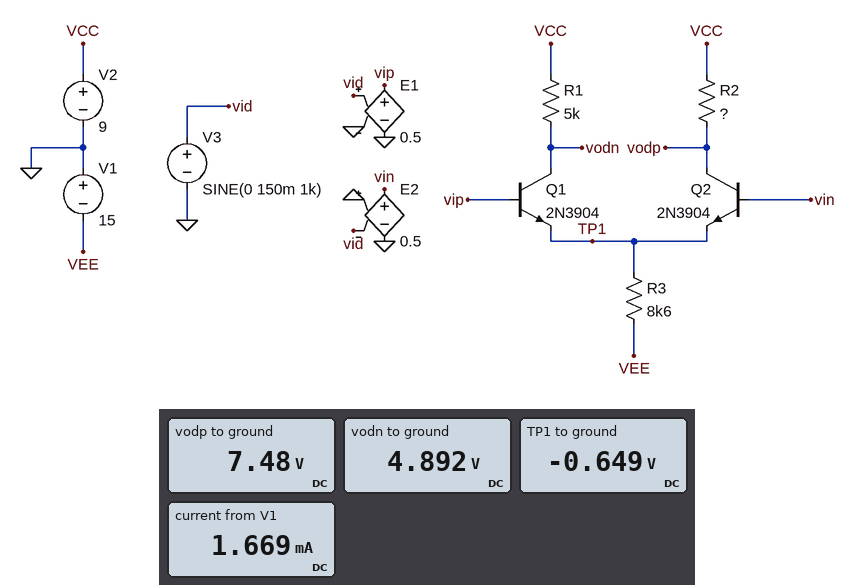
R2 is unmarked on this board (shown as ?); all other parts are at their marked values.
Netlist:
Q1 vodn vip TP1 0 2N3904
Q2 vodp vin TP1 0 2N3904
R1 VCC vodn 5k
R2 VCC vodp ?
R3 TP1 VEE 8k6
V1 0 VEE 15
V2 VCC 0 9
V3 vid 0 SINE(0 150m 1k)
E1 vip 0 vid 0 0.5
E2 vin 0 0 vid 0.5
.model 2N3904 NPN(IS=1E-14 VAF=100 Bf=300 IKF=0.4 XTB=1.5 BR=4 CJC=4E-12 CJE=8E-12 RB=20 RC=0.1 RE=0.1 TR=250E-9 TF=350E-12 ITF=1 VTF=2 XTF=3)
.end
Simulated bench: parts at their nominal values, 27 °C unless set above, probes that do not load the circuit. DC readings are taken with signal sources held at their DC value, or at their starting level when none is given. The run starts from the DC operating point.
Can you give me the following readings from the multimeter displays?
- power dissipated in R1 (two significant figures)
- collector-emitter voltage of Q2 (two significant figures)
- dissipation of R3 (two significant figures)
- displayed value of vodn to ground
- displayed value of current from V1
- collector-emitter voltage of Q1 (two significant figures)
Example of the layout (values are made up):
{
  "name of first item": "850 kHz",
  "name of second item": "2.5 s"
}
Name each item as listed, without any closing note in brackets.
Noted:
{
  "power dissipated in R1": "3.4 mW",
  "collector-emitter voltage of Q2": "8.1 V",
  "dissipation of R3": "24 mW",
  "displayed value of vodn to ground": "4.892 V",
  "displayed value of current from V1": "1.669 mA",
  "collector-emitter voltage of Q1": "5.5 V"
}
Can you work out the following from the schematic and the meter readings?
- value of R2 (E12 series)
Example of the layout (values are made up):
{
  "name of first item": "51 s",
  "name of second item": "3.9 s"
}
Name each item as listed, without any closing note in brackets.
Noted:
{
  "value of R2": "1.8 kΩ"
}
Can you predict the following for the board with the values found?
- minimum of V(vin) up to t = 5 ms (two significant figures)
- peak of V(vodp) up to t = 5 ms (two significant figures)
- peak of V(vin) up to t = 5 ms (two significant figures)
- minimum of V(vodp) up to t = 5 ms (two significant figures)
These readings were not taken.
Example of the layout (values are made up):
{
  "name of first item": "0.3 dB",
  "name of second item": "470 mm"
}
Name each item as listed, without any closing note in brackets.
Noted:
{
  "minimum of V(vin) up to t = 5 ms": "-75 mV",
  "peak of V(vodp) up to t = 5 ms": "9.0 V",
  "peak of V(vin) up to t = 5 ms": "75 mV",
  "minimum of V(vodp) up to t = 5 ms": "6.0 V"
}
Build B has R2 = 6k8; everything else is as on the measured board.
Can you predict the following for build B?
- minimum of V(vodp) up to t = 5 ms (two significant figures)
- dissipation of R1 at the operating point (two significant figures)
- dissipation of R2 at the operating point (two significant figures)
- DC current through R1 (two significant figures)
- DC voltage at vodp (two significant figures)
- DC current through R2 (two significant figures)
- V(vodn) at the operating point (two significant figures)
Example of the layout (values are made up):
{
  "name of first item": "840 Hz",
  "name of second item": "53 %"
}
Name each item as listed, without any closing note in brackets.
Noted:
{
  "minimum of V(vodp) up to t = 5 ms": "-600 mV",
  "dissipation of R1 at the operating point": "3.5 mW",
  "dissipation of R2 at the operating point": "4.6 mW",
  "DC current through R1": "840 µA",
  "DC voltage at vodp": "3.4 V",
  "DC current through R2": "830 µA",
  "V(vodn) at the operating point": "4.8 V"
}
